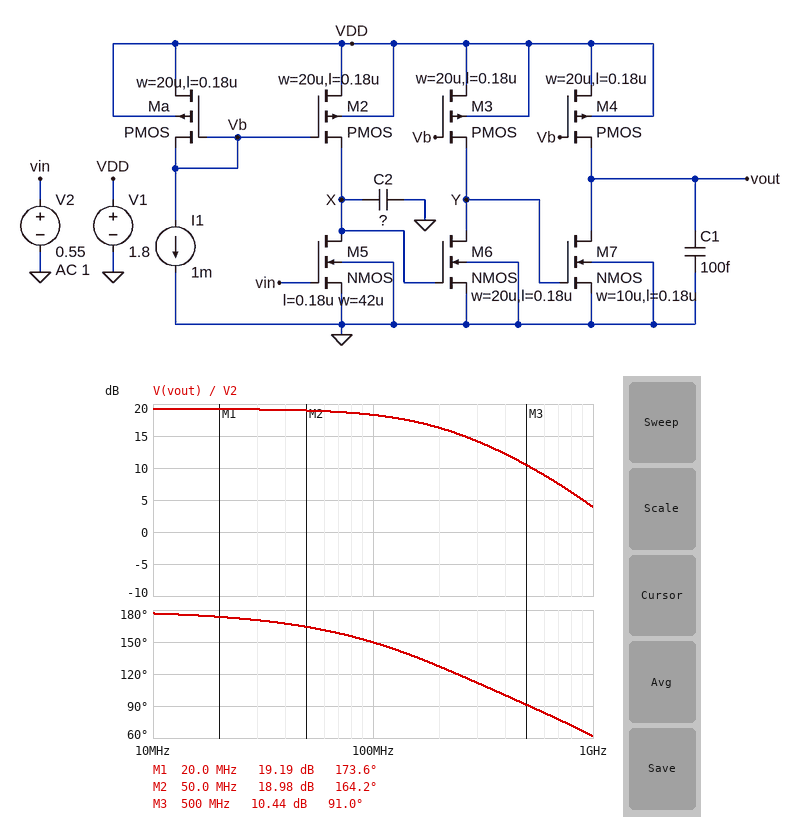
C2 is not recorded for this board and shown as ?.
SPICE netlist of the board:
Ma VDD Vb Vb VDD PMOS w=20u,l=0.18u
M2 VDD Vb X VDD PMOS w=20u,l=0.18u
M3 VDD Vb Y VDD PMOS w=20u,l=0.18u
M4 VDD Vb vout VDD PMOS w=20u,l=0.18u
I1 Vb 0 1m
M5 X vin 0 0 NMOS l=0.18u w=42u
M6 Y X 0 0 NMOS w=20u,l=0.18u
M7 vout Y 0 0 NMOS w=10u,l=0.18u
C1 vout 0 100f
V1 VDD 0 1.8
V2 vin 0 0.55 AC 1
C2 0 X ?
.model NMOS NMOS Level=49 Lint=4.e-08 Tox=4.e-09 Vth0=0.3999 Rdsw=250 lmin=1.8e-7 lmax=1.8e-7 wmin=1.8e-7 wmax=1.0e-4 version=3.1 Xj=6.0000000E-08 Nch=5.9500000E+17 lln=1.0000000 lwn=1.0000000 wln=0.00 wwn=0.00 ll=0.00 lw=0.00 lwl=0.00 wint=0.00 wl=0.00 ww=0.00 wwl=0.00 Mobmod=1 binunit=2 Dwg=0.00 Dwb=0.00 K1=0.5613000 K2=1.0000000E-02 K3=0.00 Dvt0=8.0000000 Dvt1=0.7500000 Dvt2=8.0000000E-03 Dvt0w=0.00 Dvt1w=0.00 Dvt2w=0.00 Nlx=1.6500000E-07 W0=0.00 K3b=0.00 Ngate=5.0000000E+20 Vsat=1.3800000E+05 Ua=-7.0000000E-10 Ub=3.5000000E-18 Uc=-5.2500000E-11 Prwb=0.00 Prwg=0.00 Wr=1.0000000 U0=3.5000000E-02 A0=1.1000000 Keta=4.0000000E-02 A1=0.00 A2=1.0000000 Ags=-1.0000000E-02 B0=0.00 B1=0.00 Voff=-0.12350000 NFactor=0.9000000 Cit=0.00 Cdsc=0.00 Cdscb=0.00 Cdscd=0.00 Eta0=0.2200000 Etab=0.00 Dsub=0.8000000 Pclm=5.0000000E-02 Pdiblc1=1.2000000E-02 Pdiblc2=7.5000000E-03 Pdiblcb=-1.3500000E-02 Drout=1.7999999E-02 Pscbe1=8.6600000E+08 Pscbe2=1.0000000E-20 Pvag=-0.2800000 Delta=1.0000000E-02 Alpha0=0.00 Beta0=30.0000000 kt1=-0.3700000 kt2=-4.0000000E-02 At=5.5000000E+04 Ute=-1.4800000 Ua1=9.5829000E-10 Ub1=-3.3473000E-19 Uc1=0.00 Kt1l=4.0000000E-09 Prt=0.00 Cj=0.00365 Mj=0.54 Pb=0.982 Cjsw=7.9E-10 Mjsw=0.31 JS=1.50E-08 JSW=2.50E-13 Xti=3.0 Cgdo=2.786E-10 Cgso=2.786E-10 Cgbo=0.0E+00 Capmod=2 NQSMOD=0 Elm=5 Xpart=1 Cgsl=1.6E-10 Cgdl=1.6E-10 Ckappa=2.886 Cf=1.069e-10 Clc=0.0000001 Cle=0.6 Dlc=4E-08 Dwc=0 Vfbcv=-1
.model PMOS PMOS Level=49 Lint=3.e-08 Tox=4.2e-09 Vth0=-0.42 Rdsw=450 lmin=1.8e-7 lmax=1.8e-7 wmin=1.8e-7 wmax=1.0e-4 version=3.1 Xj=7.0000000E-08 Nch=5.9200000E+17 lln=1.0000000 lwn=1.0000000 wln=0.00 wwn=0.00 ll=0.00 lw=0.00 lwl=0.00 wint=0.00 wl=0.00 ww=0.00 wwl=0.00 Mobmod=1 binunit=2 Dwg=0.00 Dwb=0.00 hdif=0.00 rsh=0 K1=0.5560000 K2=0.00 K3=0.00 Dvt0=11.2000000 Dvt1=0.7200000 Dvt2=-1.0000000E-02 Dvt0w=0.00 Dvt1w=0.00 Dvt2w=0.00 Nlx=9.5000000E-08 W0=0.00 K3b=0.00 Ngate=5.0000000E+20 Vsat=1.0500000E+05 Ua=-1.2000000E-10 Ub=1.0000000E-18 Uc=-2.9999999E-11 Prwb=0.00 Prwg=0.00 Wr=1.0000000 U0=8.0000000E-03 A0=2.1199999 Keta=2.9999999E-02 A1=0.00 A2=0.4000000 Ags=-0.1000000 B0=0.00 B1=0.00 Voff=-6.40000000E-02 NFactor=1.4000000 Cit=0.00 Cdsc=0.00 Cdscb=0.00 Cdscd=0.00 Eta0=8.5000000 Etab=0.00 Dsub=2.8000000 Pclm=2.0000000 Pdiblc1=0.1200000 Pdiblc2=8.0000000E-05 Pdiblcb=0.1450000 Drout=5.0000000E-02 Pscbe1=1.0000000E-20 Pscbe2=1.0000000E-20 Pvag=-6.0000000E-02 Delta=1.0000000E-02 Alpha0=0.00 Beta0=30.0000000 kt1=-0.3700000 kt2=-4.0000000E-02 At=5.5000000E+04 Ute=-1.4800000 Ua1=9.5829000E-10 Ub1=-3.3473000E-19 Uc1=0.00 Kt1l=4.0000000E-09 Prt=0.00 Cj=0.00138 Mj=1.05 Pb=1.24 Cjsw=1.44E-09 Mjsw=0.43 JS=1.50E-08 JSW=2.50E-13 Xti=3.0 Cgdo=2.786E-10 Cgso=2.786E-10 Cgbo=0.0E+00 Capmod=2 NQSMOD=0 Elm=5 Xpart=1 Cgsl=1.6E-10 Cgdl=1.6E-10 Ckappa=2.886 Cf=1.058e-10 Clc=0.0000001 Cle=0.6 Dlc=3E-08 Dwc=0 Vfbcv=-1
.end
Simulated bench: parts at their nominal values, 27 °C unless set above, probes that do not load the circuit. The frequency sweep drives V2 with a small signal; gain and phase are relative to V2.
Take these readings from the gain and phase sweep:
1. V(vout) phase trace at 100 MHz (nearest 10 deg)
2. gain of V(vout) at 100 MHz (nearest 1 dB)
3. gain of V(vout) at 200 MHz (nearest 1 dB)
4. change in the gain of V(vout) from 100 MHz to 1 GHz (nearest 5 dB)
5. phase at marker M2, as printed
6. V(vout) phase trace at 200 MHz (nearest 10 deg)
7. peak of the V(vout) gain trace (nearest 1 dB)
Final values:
150 deg
18 dB
16 dB
-15 dB
164.2 deg
130 deg
19 dB
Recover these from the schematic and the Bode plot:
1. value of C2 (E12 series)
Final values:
1 pF
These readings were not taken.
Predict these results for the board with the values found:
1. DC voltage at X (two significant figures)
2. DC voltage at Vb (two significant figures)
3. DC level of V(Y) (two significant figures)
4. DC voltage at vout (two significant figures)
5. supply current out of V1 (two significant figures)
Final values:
560 mV
1.1 V
1.1 V
150 mV
4.6 mA
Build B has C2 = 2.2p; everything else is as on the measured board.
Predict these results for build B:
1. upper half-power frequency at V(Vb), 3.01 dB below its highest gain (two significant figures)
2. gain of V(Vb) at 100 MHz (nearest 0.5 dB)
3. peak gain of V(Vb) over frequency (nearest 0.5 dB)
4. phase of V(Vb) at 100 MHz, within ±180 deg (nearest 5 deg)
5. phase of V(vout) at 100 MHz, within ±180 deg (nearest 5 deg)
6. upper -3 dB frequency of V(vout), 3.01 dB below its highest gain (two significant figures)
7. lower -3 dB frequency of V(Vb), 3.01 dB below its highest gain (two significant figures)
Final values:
1.5 GHz
-27.0 dB
-24.5 dB
40 deg
130 deg
100 MHz
89 MHz
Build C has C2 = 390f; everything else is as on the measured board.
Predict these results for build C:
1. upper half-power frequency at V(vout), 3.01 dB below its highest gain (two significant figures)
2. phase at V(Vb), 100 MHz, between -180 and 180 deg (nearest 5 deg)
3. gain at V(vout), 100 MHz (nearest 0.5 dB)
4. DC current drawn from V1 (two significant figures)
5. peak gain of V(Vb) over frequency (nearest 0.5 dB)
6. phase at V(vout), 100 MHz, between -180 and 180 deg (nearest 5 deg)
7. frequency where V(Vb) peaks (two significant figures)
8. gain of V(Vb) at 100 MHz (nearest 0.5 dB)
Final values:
410 MHz
70 deg
19.0 dB
4.6 mA
-13.5 dB
165 deg
760 MHz
-24.0 dB
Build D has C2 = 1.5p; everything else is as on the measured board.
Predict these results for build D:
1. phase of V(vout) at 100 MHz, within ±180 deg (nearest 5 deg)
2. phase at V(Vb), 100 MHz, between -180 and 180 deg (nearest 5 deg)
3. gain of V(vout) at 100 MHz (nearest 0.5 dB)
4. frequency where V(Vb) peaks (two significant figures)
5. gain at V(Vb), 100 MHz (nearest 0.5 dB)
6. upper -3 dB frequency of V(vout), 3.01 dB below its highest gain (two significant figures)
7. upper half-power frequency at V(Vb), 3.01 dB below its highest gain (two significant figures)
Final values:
140 deg
50 deg
17.5 dB
450 MHz
-25.5 dB
140 MHz
1.6 GHz
